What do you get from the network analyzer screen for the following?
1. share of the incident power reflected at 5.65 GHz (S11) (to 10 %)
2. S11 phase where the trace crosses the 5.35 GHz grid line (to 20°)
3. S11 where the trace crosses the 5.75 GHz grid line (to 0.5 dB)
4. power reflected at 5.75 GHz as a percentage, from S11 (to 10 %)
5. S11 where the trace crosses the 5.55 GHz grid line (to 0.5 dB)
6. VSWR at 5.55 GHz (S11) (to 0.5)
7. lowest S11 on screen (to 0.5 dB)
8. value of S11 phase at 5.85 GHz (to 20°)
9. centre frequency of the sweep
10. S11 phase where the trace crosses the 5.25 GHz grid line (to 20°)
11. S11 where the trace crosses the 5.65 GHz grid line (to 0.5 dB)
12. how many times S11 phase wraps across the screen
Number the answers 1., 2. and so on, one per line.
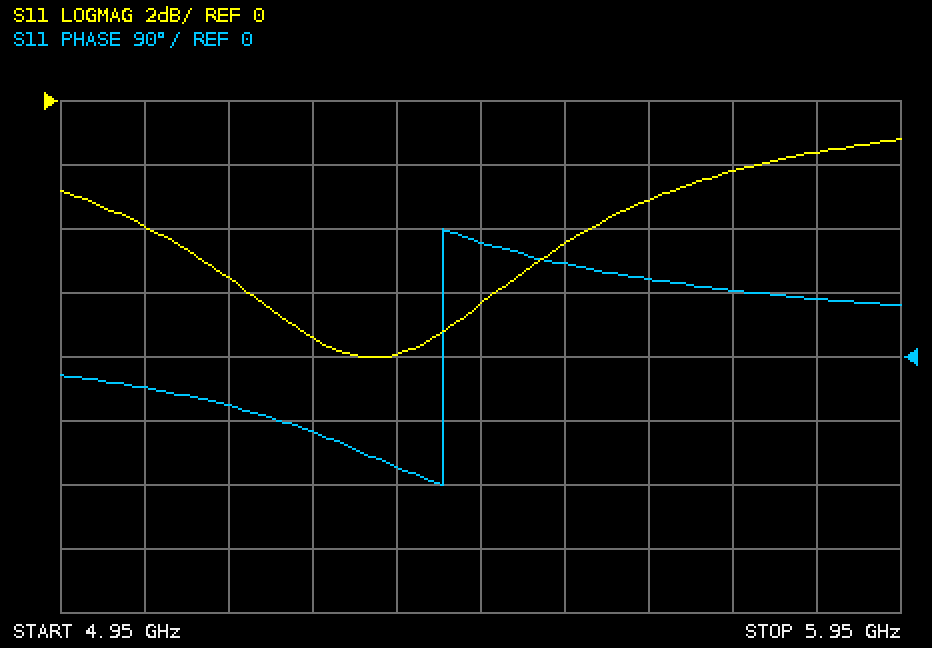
1. 50 %
2. -160°
3. -2.0 dB
4. 60 %
5. -4.5 dB
6. 4.0
7. -8.0 dB
8. 80°
9. 5.45 GHz
10. -100°
11. -3.0 dB
12. 1
